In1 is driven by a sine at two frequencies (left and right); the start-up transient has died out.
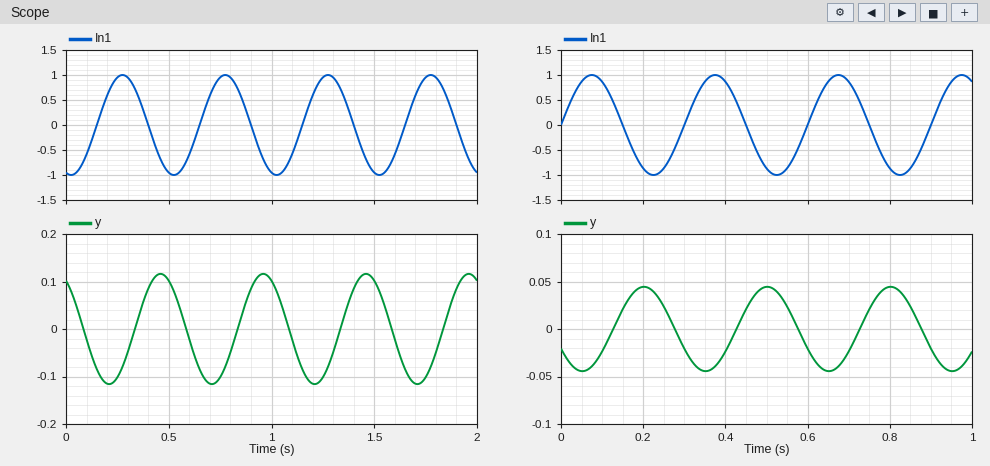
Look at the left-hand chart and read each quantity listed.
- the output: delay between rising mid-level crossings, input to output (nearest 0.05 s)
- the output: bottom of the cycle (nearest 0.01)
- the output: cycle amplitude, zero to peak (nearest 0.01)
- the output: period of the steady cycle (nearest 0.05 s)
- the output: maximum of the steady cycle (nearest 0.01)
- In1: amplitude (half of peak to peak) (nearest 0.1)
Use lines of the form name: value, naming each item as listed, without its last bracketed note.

the output: delay between rising mid-level crossings, input to output: 0.20 s
the output: bottom of the cycle: -0.12
the output: cycle amplitude, zero to peak: 0.12
the output: period of the steady cycle: 0.50 s
the output: maximum of the steady cycle: 0.12
In1: amplitude (half of peak to peak): 1.0
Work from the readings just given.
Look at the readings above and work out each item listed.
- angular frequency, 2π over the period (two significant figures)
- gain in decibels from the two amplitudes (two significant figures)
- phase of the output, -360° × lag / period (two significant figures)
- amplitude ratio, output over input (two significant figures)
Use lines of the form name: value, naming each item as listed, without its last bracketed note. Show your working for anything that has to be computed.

angular frequency, 2π over the period: 2π / 0.5 = 13 rad/s
gain in decibels from the two amplitudes: 20 log10(0.12 / 1) = -18 dB
phase of the output, -360° × lag / period: -360 × 0.2 / 0.5 = -140°
amplitude ratio, output over input: 0.12 / 1 = 0.12
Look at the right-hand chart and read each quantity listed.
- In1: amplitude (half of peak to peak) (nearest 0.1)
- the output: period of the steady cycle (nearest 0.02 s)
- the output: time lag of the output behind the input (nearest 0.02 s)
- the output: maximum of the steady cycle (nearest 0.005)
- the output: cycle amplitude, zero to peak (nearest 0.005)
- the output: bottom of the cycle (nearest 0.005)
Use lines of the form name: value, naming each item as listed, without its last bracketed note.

In1: amplitude (half of peak to peak): 1.0
the output: period of the steady cycle: 0.30 s
the output: time lag of the output behind the input: 0.12 s
the output: maximum of the steady cycle: 0.045
the output: cycle amplitude, zero to peak: 0.045
the output: bottom of the cycle: -0.045
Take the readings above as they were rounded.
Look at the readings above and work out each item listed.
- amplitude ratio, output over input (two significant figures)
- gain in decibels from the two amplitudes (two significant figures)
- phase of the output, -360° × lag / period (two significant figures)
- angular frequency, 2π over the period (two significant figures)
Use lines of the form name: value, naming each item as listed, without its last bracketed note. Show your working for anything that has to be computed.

amplitude ratio, output over input: 0.045 / 1 = 0.045
gain in decibels from the two amplitudes: 20 log10(0.045 / 1) = -27 dB
phase of the output, -360° × lag / period: -360 × 0.12 / 0.3 = -140°
angular frequency, 2π over the period: 2π / 0.3 = 21 rad/s
